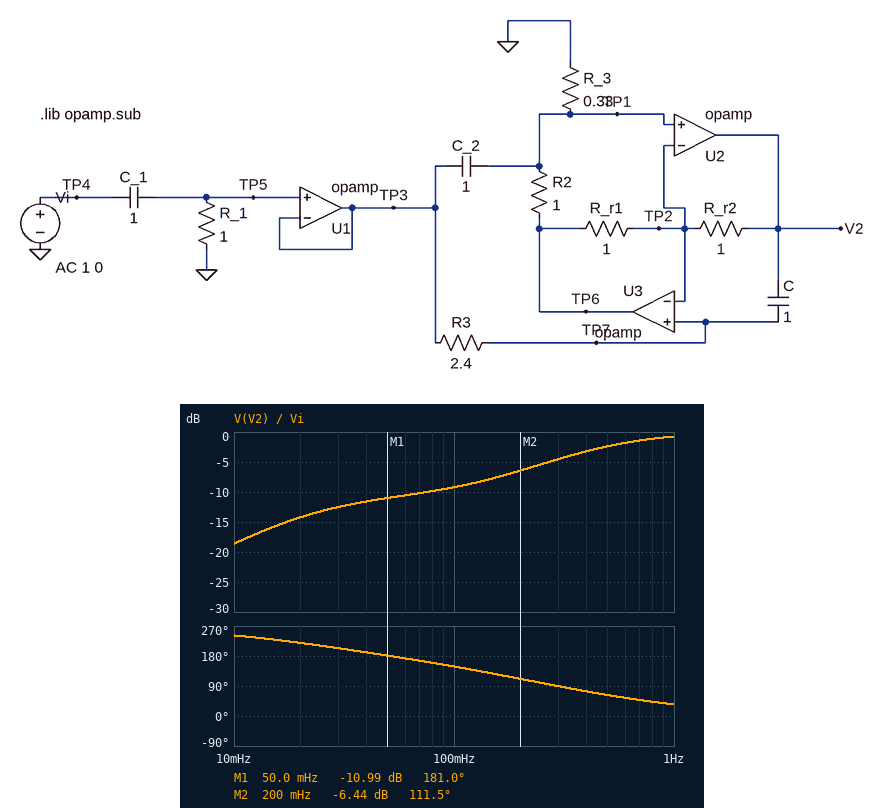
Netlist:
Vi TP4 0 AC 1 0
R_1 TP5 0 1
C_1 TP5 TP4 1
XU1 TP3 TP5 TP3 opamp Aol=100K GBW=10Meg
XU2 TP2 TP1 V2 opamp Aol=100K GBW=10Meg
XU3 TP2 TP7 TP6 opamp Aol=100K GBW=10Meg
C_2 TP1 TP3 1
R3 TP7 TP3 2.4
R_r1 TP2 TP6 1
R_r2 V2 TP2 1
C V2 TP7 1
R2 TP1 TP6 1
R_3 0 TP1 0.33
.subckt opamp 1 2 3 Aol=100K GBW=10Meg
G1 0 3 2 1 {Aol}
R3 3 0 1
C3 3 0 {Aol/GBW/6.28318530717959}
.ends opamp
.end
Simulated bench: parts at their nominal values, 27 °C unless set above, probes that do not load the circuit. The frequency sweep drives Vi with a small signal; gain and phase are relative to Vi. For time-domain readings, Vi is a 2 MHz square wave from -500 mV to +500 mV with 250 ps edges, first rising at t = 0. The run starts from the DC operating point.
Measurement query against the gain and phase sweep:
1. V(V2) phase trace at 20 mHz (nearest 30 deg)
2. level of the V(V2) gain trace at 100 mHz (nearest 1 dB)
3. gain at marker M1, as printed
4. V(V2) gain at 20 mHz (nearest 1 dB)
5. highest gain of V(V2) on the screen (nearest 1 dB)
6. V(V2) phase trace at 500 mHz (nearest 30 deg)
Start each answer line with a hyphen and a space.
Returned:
- 210 deg
- -9 dB
- -10.99 dB
- -14 dB
- -1 dB
- 60 deg
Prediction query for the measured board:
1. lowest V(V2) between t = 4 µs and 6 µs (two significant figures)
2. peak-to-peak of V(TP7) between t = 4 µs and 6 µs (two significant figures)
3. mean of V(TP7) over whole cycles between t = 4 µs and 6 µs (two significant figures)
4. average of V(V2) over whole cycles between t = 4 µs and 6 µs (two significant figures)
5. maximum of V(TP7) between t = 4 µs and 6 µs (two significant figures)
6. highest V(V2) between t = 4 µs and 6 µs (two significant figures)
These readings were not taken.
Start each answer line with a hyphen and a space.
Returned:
- -140 mV
- 1.3 V
- 500 mV
- 500 mV
- 1.1 V
- 1.1 V
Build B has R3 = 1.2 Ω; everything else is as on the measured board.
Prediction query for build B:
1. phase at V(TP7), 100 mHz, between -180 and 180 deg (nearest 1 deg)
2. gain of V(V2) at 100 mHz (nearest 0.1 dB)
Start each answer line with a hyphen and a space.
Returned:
- -19 deg
- -4.9 dB
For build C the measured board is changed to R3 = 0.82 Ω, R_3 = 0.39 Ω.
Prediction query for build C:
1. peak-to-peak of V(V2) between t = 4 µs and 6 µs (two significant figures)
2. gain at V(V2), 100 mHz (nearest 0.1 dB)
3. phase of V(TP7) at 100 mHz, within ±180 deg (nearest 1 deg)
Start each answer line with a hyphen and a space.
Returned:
- 1.3 V
- -3.4 dB
- -5 deg
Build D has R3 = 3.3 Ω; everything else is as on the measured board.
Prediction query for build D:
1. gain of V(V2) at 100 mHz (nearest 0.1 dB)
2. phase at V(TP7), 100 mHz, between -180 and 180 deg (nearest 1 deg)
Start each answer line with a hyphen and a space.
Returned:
- -11.0 dB
- 145 deg
